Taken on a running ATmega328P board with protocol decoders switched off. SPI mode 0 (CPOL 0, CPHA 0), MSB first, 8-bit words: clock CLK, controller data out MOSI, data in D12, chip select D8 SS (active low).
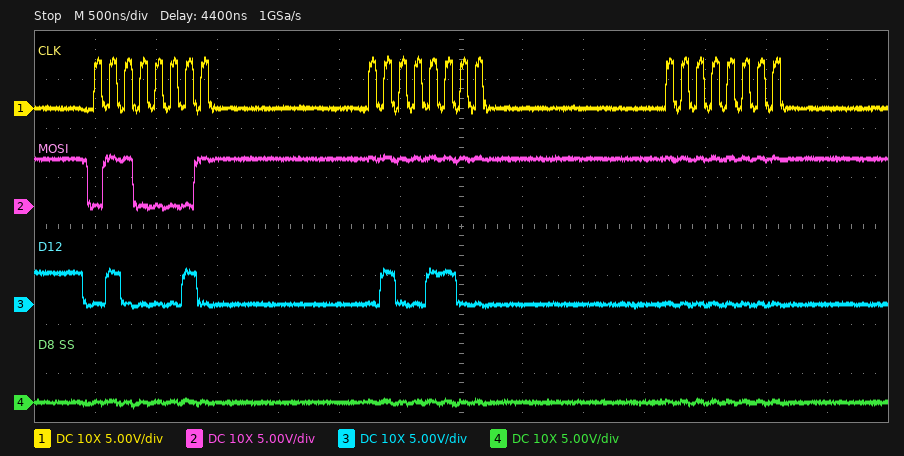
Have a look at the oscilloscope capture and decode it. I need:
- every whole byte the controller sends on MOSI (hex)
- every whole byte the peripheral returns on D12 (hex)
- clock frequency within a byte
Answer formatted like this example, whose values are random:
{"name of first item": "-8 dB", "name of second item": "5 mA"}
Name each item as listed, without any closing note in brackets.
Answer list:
{"every whole byte the controller sends on MOSI": "61 FF FF", "every whole byte the peripheral returns on D12": "42 4C 00", "clock frequency within a byte": "8 MHz"}
